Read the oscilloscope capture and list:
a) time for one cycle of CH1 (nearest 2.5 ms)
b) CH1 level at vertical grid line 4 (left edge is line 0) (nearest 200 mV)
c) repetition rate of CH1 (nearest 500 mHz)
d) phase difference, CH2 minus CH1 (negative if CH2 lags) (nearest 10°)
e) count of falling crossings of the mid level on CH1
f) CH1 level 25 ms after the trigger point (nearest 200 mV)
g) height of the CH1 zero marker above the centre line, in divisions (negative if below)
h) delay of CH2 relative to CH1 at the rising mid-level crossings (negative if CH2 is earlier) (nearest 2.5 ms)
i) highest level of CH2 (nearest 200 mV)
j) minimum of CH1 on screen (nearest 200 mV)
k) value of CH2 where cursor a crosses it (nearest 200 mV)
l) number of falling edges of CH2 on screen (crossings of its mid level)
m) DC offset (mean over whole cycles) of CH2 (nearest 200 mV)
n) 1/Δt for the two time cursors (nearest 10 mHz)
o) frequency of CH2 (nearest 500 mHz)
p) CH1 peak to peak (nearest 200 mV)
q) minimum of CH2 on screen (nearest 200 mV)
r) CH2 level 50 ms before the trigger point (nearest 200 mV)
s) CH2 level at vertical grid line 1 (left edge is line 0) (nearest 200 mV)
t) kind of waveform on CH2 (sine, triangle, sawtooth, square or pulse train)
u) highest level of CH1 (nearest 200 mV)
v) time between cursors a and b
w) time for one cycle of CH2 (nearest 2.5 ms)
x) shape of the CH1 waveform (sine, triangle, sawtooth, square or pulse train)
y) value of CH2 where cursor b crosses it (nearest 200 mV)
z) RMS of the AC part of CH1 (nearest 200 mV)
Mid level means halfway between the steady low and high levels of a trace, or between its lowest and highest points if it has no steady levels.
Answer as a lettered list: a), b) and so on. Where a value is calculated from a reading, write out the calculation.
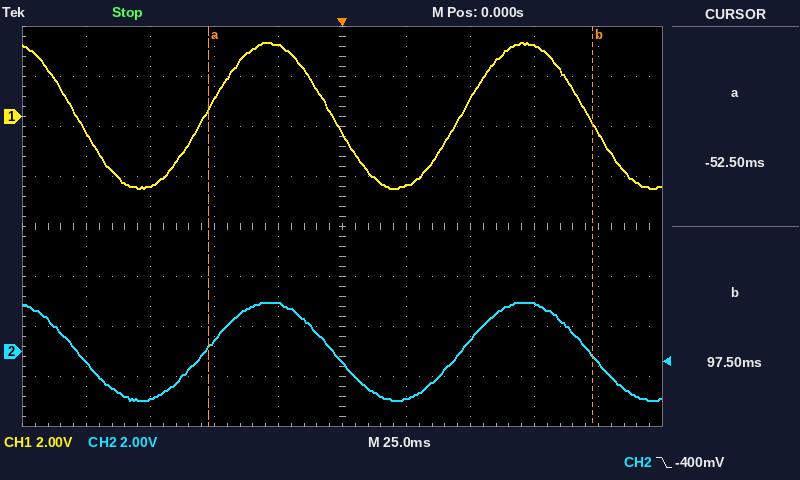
a) 100.0 ms
b) 2.8 V
c) 1 / 100.0 ms ≈ 10.0 Hz
d) −360° × (0.0 ms) / 100.0 ms ≈ 0°
e) 3
f) -2.8 V
g) +2.2 div
h) 0.0 ms
i) 2.0 V
j) -2.8 V
k) 200 mV
l) 3
m) (2.0 V + (-2.0 V)) / 2 ≈ 0.0 V
n) 1 / 150.0 ms ≈ 6.67 Hz
o) 1 / 100.0 ms ≈ 10.0 Hz
p) 3.0 V − (-2.8 V) = 5.8 V
q) -2.0 V
r) 400 mV
s) -400 mV
t) sine
u) 3.0 V
v) 97.5 ms − (-52.5 ms) = 150.0 ms
w) 100.0 ms
x) sine
y) -200 mV
z) 5.8 V / (2√2) ≈ 2.0 V
